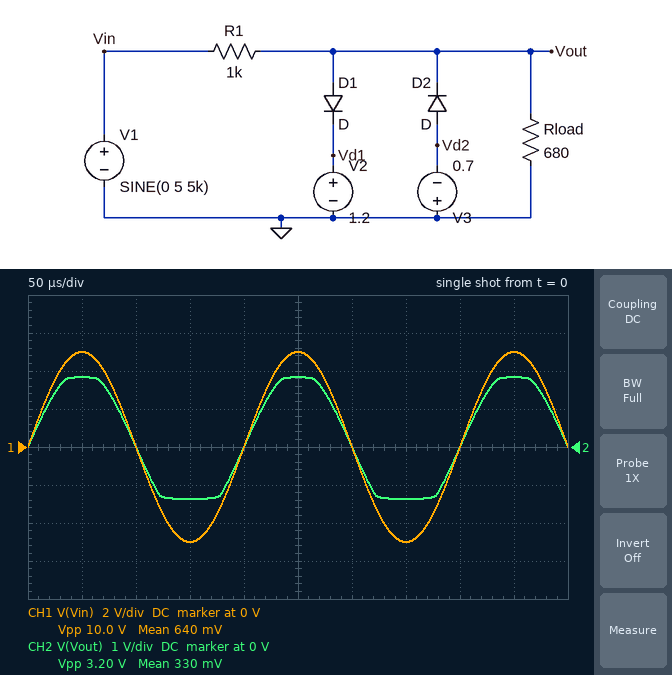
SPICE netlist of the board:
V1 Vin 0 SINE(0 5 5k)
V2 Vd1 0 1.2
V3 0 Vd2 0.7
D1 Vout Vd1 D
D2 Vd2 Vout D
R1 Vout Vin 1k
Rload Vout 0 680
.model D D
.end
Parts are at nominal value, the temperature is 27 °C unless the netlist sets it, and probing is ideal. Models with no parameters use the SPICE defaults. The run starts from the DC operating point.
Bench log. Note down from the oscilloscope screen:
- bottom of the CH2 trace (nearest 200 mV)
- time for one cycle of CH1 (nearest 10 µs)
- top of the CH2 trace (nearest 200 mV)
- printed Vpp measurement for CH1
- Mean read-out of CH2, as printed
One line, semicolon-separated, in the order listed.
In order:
-1.4 V; 200 µs; 1.8 V; 10.0 V; 330 mV
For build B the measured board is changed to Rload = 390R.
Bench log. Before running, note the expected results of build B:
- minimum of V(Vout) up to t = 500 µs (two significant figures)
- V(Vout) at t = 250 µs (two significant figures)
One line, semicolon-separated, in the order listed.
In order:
-1.3 V; 1.4 V
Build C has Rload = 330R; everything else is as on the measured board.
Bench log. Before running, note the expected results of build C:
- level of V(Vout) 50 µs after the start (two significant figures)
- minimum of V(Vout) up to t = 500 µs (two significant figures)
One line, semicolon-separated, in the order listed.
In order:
1.2 V; -1.2 V
